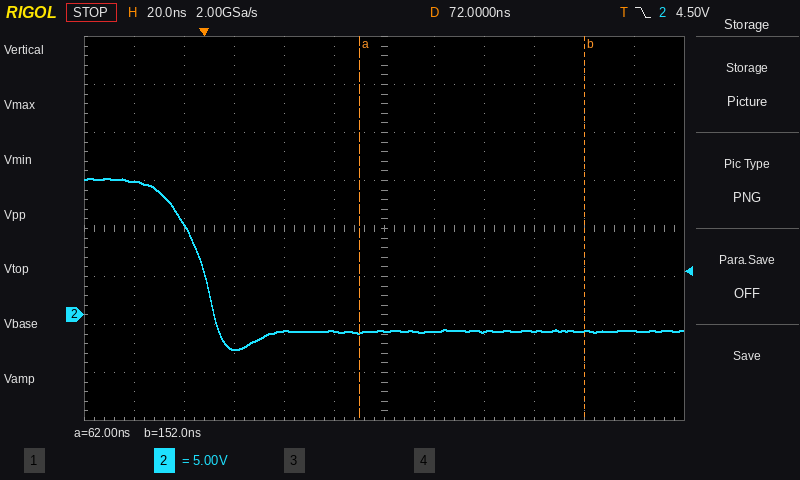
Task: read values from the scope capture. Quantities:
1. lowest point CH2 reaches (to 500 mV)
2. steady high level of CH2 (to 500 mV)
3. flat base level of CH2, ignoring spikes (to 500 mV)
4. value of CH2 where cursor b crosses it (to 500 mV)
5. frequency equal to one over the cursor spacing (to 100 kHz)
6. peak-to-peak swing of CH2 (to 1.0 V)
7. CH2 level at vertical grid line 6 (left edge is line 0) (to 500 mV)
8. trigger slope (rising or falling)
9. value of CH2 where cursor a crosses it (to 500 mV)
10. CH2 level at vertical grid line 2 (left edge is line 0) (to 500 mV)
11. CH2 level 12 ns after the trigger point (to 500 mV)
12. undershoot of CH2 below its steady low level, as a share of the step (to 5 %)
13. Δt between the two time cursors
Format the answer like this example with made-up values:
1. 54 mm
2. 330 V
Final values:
1. -3.5 V
2. 14.0 V
3. -1.5 V
4. -1.5 V
5. 11.1 MHz
6. 18.0 V
7. -1.5 V
8. falling
9. -2.0 V
10. 9.5 V
11. -3.5 V
12. 10 %
13. 90 ns
